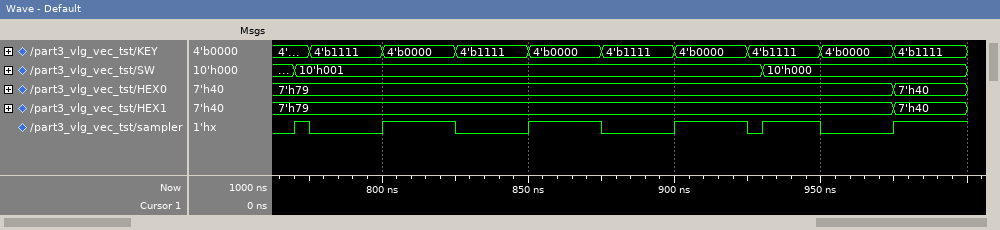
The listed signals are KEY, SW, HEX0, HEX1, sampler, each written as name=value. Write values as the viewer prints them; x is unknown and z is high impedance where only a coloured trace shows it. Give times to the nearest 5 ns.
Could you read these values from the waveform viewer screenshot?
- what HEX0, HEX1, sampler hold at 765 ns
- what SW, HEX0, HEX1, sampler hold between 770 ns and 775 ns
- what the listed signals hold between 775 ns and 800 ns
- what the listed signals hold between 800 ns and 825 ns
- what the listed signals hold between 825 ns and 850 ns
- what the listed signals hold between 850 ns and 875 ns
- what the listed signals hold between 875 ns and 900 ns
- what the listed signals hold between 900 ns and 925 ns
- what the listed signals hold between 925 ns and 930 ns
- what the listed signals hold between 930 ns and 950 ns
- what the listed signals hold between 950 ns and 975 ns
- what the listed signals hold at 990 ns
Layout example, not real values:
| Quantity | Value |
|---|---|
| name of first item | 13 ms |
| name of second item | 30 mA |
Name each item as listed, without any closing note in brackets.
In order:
| Quantity | Value |
|---|---|
| what HEX0, HEX1, sampler hold at 765 ns | HEX0=7'h79, HEX1=7'h79, sampler=0 |
| what SW, HEX0, HEX1, sampler hold between 770 ns and 775 ns | SW=10'h001, HEX0=7'h79, HEX1=7'h79, sampler=1 |
| what the listed signals hold between 775 ns and 800 ns | KEY=4'b1111, SW=10'h001, HEX0=7'h79, HEX1=7'h79, sampler=0 |
| what the listed signals hold between 800 ns and 825 ns | KEY=4'b0000, SW=10'h001, HEX0=7'h79, HEX1=7'h79, sampler=1 |
| what the listed signals hold between 825 ns and 850 ns | KEY=4'b1111, SW=10'h001, HEX0=7'h79, HEX1=7'h79, sampler=0 |
| what the listed signals hold between 850 ns and 875 ns | KEY=4'b0000, SW=10'h001, HEX0=7'h79, HEX1=7'h79, sampler=1 |
| what the listed signals hold between 875 ns and 900 ns | KEY=4'b1111, SW=10'h001, HEX0=7'h79, HEX1=7'h79, sampler=0 |
| what the listed signals hold between 900 ns and 925 ns | KEY=4'b0000, SW=10'h001, HEX0=7'h79, HEX1=7'h79, sampler=1 |
| what the listed signals hold between 925 ns and 930 ns | KEY=4'b1111, SW=10'h001, HEX0=7'h79, HEX1=7'h79, sampler=0 |
| what the listed signals hold between 930 ns and 950 ns | KEY=4'b1111, SW=10'h000, HEX0=7'h79, HEX1=7'h79, sampler=1 |
| what the listed signals hold between 950 ns and 975 ns | KEY=4'b0000, SW=10'h000, HEX0=7'h79, HEX1=7'h79, sampler=0 |
| what the listed signals hold at 990 ns | KEY=4'b1111, SW=10'h000, HEX0=7'h40, HEX1=7'h40, sampler=1 |
